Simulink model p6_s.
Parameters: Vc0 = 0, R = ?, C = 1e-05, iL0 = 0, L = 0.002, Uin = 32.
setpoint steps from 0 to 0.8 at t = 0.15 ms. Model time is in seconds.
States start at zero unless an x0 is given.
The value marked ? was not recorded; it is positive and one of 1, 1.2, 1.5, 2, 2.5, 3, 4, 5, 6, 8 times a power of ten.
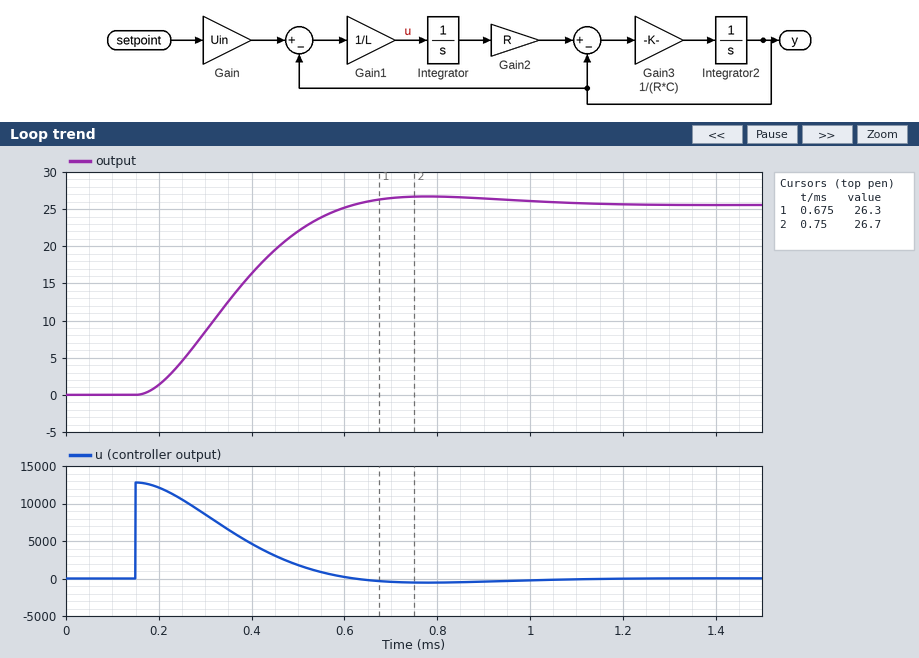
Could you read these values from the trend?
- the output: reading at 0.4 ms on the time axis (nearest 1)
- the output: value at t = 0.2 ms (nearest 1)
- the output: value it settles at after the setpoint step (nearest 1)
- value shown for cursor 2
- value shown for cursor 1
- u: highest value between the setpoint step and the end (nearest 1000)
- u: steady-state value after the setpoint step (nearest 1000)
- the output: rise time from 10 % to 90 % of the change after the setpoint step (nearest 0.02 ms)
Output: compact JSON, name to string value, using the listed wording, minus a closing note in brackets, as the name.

{"the output: reading at 0.4 ms on the time axis": "16", "the output: value at t = 0.2 ms": "1", "the output: value it settles at after the setpoint step": "26", "value shown for cursor 2": "26.7", "value shown for cursor 1": "26.3", "u: highest value between the setpoint step and the end": "13000", "u: steady-state value after the setpoint step": "0", "the output: rise time from 10 % to 90 % of the change after the setpoint step": "0.30 ms"}
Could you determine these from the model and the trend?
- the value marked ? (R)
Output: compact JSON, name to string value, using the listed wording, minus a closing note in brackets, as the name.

{"the value marked ?": "10"}
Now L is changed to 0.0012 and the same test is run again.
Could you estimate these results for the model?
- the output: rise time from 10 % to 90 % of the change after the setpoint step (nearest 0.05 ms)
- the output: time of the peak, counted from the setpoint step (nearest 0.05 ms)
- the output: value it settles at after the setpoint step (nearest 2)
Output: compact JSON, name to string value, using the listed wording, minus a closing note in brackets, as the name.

{"the output: rise time from 10 % to 90 % of the change after the setpoint step": "0.20 ms", "the output: time of the peak, counted from the setpoint step": "0.40 ms", "the output: value it settles at after the setpoint step": "26"}
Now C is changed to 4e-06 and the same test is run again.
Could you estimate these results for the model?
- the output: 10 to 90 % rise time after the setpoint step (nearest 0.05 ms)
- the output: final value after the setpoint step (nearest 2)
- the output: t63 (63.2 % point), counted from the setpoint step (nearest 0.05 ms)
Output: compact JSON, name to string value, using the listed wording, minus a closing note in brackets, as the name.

{"the output: 10 to 90 % rise time after the setpoint step": "0.35 ms", "the output: final value after the setpoint step": "26", "the output: t63 (63.2 % point), counted from the setpoint step": "0.20 ms"}
